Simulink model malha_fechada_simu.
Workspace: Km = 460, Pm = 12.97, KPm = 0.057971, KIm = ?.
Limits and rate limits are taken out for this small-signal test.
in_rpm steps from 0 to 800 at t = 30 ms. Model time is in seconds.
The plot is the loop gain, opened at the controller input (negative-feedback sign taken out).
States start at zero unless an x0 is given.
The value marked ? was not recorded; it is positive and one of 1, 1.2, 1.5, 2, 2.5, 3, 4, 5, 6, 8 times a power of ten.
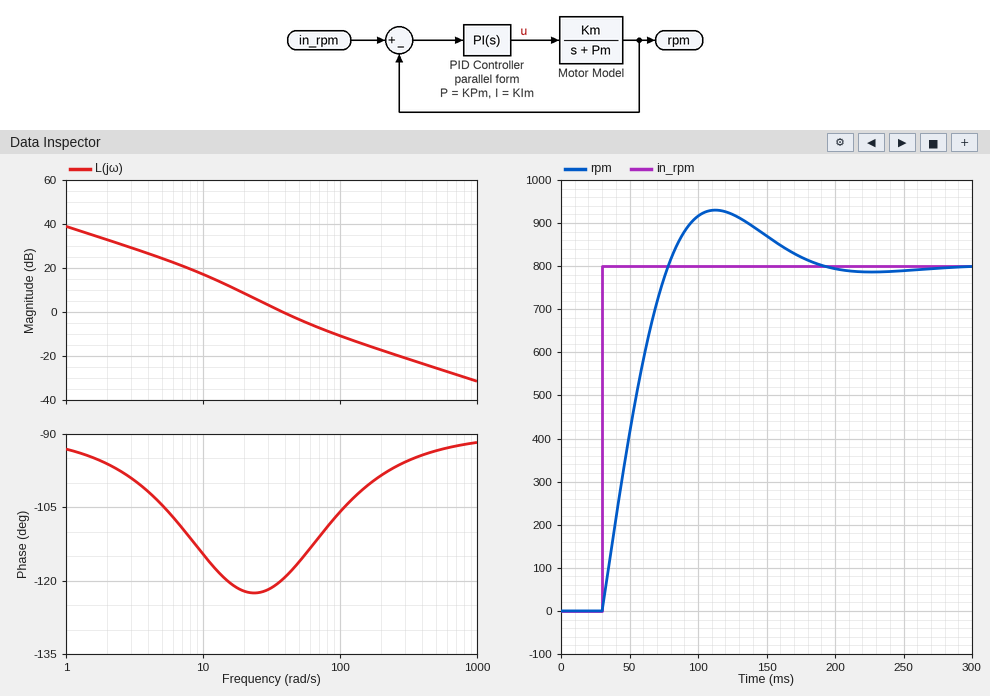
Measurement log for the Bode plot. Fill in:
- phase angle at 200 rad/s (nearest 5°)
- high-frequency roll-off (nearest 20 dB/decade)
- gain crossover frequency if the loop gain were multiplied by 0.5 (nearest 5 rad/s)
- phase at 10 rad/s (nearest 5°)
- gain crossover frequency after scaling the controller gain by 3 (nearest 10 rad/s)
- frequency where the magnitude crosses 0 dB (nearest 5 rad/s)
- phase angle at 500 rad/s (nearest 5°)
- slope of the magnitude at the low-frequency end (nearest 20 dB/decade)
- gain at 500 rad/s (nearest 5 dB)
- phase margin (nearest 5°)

-100°
-20 dB/decade
25 rad/s
-115°
90 rad/s
40 rad/s
-95°
-20 dB/decade
-25 dB
60°
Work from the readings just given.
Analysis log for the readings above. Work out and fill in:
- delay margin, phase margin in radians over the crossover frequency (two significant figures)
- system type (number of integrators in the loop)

0.026 s
1
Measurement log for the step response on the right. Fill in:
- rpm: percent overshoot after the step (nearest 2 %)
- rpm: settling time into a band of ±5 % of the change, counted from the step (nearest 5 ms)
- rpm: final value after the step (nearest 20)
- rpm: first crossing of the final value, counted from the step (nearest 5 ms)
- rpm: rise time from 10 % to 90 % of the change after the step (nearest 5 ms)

16 %
135 ms
800
50 ms
35 ms
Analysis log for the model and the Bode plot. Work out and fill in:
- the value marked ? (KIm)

2.5
